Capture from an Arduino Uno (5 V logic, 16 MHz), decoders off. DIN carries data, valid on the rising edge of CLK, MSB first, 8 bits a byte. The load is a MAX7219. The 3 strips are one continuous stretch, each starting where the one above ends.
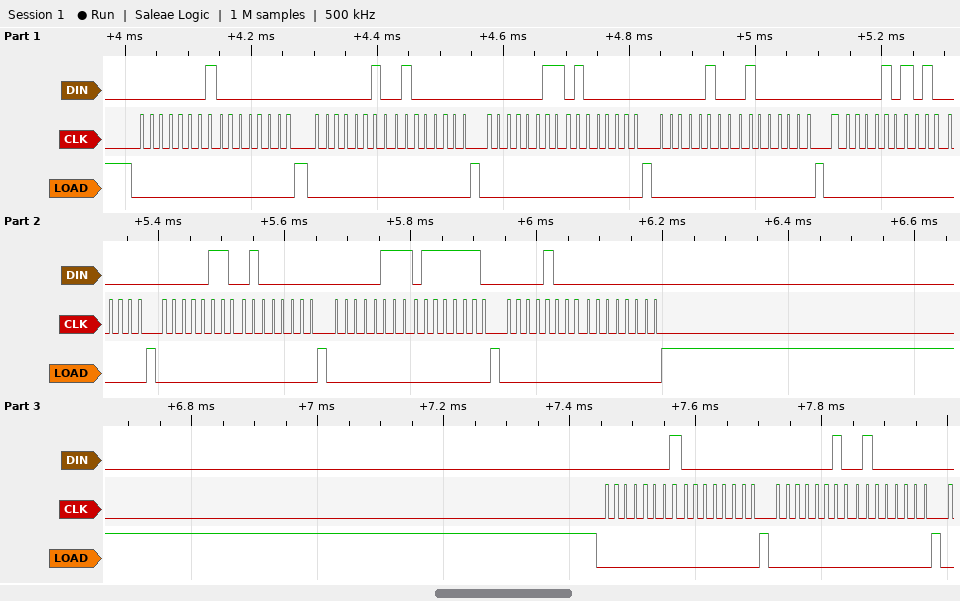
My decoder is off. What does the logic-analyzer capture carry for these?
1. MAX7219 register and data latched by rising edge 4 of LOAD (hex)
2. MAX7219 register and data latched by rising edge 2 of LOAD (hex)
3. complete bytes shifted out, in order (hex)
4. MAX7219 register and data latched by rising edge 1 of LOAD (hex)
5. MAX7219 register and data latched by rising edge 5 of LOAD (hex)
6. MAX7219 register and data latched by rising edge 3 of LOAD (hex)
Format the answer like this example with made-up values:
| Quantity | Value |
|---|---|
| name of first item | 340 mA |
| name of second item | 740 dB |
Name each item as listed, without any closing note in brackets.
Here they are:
| Quantity | Value |
|---|---|
| MAX7219 register and data latched by rising edge 4 of LOAD | register 0x4, data 0x40 |
| MAX7219 register and data latched by rising edge 2 of LOAD | register 0x2, data 0x40 |
| complete bytes shifted out, in order | 0x01 0x00 0x02 0x40 0x03 0x40 0x04 0x40 0x05 0x40 0x06 0x40 0x07 0x7E 0x08 0x00 0x01 0x00 0x02 0x40 |
| MAX7219 register and data latched by rising edge 1 of LOAD | register 0x1, data 0x00 |
| MAX7219 register and data latched by rising edge 5 of LOAD | register 0x5, data 0x40 |
| MAX7219 register and data latched by rising edge 3 of LOAD | register 0x3, data 0x40 |
